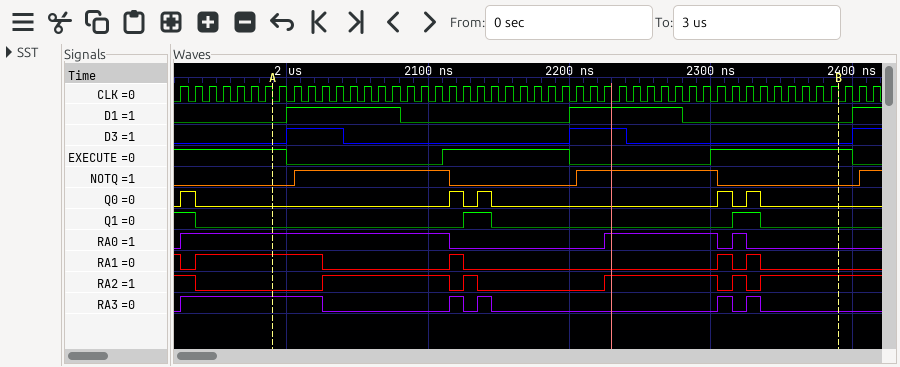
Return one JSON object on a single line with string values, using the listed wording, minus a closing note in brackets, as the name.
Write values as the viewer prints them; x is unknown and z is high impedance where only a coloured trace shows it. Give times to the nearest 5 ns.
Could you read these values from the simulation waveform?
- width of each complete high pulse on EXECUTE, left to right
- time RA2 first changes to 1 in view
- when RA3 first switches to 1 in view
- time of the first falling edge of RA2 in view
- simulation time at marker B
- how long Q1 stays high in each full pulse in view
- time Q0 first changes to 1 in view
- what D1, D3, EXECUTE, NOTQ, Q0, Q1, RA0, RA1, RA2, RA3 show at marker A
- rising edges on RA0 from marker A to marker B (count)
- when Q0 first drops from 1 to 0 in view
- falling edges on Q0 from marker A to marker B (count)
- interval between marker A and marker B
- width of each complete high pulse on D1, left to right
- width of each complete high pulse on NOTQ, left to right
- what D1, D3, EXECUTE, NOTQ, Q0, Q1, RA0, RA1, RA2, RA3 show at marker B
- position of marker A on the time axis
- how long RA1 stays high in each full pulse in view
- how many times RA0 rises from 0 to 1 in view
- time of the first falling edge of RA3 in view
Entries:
{"width of each complete high pulse on EXECUTE, left to right": "90 ns, 100 ns", "time RA2 first changes to 1 in view": "2025 ns", "when RA3 first switches to 1 in view": "1925 ns", "time of the first falling edge of RA2 in view": "1935 ns", "simulation time at marker B": "2390 ns", "how long Q1 stays high in each full pulse in view": "20 ns, 20 ns", "time Q0 first changes to 1 in view": "1925 ns", "what D1, D3, EXECUTE, NOTQ, Q0, Q1, RA0, RA1, RA2, RA3 show at marker A": "D1=0, D3=0, EXECUTE=1, NOTQ=0, Q0=0, Q1=0, RA0=1, RA1=1, RA2=0, RA3=1", "rising edges on RA0 from marker A to marker B": "2", "when Q0 first drops from 1 to 0 in view": "1935 ns", "falling edges on Q0 from marker A to marker B": "4", "interval between marker A and marker B": "400 ns", "width of each complete high pulse on D1, left to right": "80 ns, 80 ns", "width of each complete high pulse on NOTQ, left to right": "110 ns, 100 ns", "what D1, D3, EXECUTE, NOTQ, Q0, Q1, RA0, RA1, RA2, RA3 show at marker B": "D1=0, D3=0, EXECUTE=1, NOTQ=0, Q0=0, Q1=0, RA0=0, RA1=0, RA2=1, RA3=0", "position of marker A on the time axis": "1990 ns", "how long RA1 stays high in each full pulse in view": "90 ns, 10 ns, 10 ns, 10 ns", "how many times RA0 rises from 0 to 1 in view": "3", "time of the first falling edge of RA3 in view": "2025 ns"}
